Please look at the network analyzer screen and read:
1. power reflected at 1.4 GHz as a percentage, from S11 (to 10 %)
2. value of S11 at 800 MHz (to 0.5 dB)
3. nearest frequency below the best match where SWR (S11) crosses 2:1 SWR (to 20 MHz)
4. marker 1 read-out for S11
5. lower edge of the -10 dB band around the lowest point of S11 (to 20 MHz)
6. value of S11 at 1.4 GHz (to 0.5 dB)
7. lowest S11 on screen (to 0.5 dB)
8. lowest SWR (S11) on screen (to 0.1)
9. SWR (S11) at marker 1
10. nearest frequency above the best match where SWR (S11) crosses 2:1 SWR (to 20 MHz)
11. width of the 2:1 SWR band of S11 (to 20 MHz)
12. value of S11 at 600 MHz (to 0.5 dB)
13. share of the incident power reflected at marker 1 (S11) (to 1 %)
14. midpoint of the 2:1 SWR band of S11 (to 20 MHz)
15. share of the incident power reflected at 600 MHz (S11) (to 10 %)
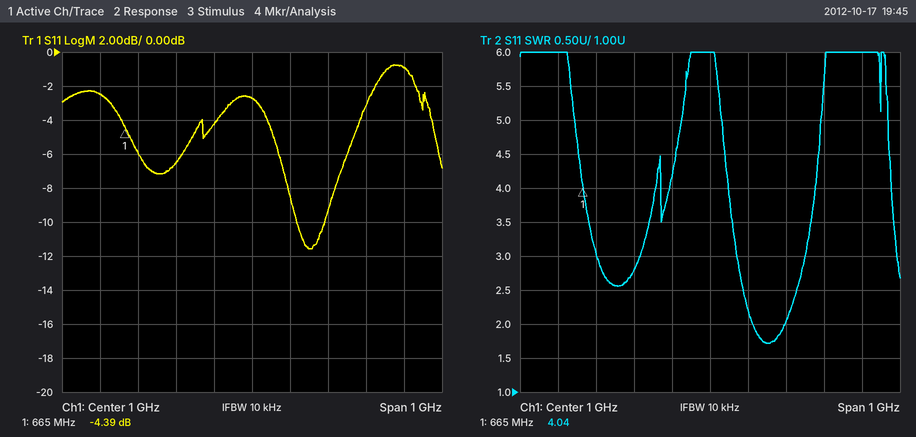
80 %
-6.5 dB
1.12 GHz
-4.39 dB
1.12 GHz
-1.0 dB
-11.5 dB
1.7
4.04
1.20 GHz
80 MHz
-2.5 dB
36 %
1.16 GHz
60 %
